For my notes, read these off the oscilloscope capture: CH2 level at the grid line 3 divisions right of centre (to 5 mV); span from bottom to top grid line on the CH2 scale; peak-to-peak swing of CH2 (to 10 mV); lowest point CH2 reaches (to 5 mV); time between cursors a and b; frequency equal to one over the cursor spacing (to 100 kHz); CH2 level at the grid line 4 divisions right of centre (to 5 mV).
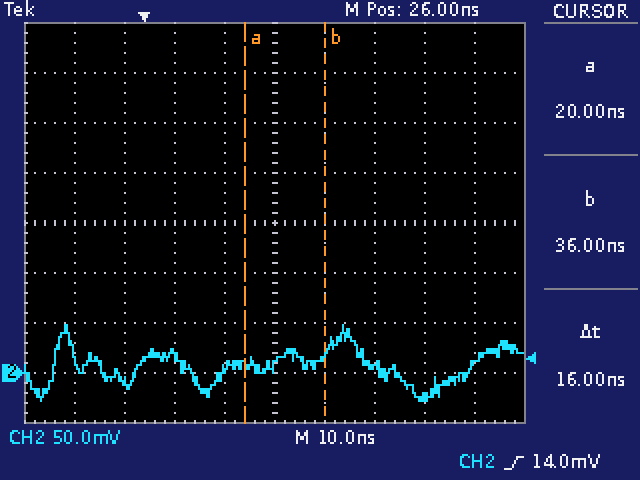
-25 mV
400 mV
80 mV
-30 mV
16 ns
62.5 MHz
10 mV
